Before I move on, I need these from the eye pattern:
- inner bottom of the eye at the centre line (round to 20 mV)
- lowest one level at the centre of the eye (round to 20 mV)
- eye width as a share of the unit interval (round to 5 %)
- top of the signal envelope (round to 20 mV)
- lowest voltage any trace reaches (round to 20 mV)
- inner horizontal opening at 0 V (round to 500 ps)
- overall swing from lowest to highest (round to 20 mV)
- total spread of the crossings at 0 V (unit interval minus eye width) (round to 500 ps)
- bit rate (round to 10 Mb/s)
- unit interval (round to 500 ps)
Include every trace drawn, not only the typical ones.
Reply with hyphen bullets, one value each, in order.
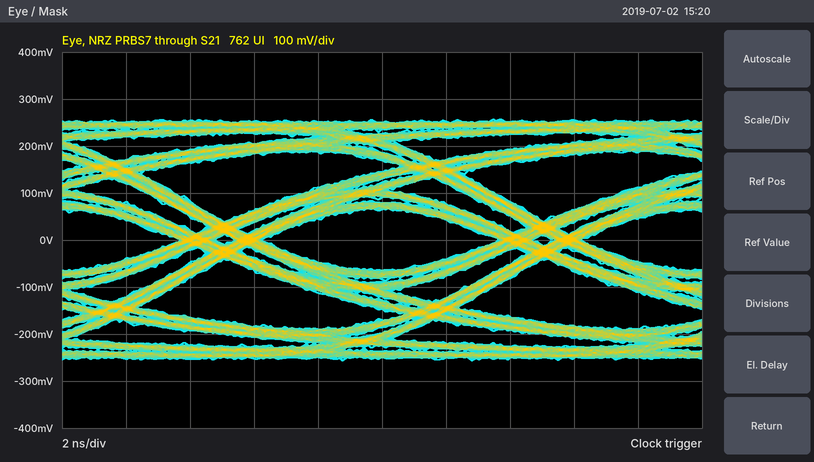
- -60 mV
- 60 mV
- 75 %
- 260 mV
- -260 mV
- 7.5 ns
- 520 mV
- 2.5 ns
- 100 Mb/s
- 10.0 ns
